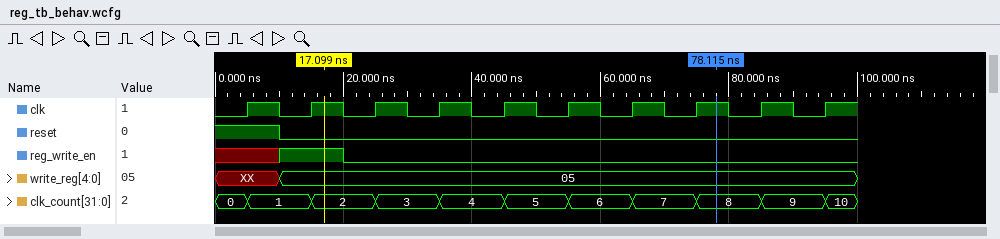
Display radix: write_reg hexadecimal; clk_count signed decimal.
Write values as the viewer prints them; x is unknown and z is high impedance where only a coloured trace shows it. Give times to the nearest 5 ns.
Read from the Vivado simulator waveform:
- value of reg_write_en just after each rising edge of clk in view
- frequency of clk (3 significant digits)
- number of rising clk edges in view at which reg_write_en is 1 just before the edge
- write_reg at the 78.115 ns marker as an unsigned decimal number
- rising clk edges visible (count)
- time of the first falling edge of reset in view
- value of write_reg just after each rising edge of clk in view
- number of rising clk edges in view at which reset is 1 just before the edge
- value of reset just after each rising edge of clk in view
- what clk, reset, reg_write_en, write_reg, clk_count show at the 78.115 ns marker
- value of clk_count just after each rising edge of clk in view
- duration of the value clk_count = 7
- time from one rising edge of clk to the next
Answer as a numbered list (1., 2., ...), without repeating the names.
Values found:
1. x 1 0 0 0 0 0 0 0 0
2. 100 MHz
3. 1
4. 5
5. 10
6. 10 ns
7. XX, 05, 05, 05, 05, 05, 05, 05, 05, 05
8. 1
9. 1 0 0 0 0 0 0 0 0 0
10. clk=1, reset=0, reg_write_en=0, write_reg=05, clk_count=8
11. 1, 2, 3, 4, 5, 6, 7, 8, 9, 10
12. 10 ns
13. 10 ns
